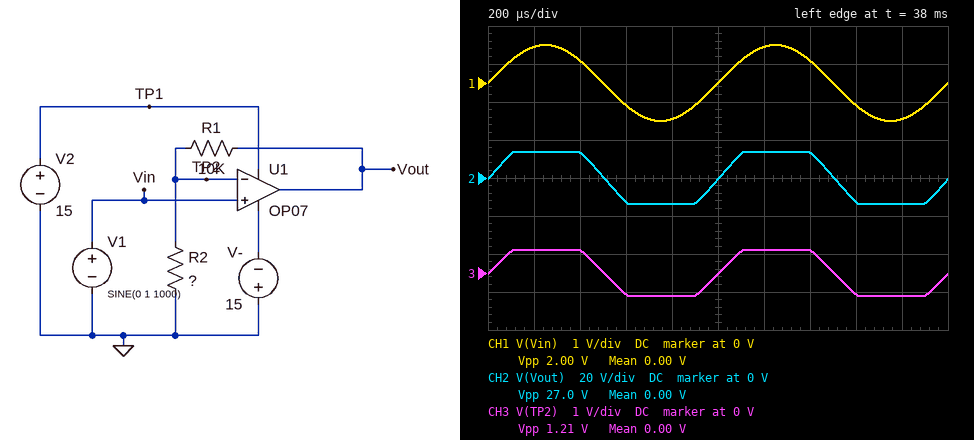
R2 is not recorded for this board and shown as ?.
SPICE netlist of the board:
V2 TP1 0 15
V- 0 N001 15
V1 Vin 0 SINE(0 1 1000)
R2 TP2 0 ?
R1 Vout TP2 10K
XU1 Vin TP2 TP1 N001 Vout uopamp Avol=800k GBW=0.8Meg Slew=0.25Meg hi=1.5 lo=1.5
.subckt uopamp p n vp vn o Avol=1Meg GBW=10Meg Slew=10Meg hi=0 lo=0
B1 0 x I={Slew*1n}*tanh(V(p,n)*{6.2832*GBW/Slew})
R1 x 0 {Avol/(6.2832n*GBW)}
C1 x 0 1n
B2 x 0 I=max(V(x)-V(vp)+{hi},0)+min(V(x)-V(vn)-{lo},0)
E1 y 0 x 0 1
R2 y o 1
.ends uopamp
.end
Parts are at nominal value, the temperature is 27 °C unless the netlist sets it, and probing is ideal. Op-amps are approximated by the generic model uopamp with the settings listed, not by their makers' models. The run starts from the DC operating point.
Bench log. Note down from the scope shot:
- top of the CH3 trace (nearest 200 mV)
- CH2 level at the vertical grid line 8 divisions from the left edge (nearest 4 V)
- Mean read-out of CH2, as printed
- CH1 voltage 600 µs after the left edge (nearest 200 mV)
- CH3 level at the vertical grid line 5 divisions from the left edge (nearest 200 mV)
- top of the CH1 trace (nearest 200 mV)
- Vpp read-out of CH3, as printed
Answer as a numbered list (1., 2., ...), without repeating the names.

1. 600 mV
2. -12 V
3. 0.00 V
4. -600 mV
5. 0 V
6. 1.0 V
7. 1.21 V
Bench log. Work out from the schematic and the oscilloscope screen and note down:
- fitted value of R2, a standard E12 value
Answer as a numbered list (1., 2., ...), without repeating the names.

1. 470 Ω
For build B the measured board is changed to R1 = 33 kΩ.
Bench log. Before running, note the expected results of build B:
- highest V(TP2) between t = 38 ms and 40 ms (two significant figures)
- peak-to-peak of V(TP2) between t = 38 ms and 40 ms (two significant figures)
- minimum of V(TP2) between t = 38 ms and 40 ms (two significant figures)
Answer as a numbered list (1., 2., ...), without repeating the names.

1. 190 mV
2. 380 mV
3. -190 mV
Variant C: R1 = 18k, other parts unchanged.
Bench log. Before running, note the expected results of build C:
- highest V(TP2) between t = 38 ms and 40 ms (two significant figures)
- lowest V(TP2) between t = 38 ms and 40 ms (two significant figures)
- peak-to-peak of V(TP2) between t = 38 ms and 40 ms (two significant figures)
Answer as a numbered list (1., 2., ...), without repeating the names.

1. 340 mV
2. -340 mV
3. 690 mV
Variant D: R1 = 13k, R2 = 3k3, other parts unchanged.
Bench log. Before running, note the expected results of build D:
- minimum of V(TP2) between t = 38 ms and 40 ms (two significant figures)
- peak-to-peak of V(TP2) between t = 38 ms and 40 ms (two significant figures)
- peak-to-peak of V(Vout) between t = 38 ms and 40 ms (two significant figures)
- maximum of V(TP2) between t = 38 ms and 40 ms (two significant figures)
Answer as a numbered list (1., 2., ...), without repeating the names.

1. -1.0 V
2. 2.0 V
3. 9.9 V
4. 1.0 V
